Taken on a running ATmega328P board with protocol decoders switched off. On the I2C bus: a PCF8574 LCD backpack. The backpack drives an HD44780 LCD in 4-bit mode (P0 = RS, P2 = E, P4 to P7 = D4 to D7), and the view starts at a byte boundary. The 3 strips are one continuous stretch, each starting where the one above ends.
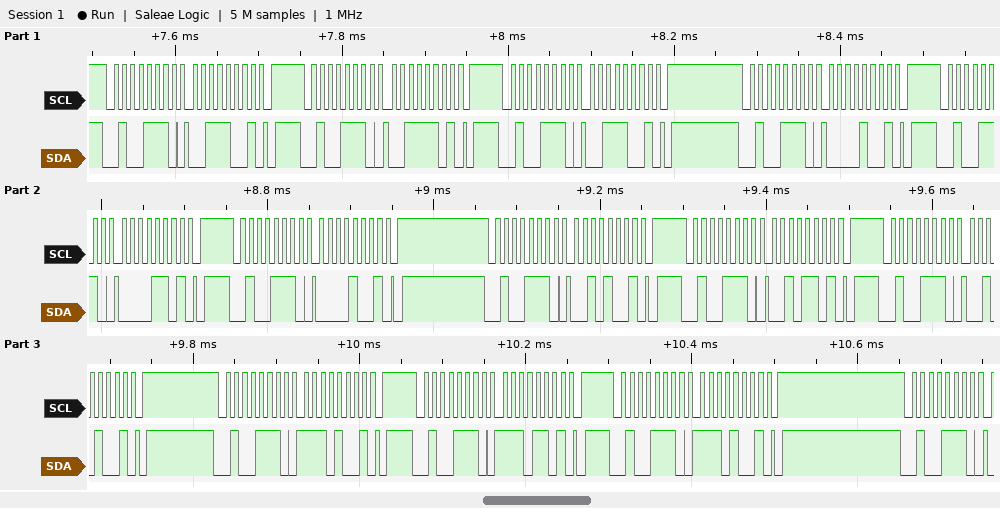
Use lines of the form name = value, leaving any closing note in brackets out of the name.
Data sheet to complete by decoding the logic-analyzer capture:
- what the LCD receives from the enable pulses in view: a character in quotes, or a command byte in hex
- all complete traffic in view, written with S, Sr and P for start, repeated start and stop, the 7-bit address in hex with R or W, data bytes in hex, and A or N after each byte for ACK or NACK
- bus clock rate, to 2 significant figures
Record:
what the LCD receives from the enable pulses in view: a character in quotes, or a command byte in hex = '0' '.'
all complete traffic in view, written with S, Sr and P for start, repeated start and stop, the 7-bit address in hex with R or W, data bytes in hex, and A or N after each byte for ACK or NACK = S 27W A 39 A P S 27W A 3D A P S 27W A 39 A P S 27W A 09 A P S 27W A 0D A P S 27W A 09 A P S 27W A 29 A P S 27W A 2D A P S 27W A 29 A P S 27W A E9 A P S 27W A ED A P S 27W A E9 A P S 27W A
bus clock rate, to 2 significant figures = 100 kHz
